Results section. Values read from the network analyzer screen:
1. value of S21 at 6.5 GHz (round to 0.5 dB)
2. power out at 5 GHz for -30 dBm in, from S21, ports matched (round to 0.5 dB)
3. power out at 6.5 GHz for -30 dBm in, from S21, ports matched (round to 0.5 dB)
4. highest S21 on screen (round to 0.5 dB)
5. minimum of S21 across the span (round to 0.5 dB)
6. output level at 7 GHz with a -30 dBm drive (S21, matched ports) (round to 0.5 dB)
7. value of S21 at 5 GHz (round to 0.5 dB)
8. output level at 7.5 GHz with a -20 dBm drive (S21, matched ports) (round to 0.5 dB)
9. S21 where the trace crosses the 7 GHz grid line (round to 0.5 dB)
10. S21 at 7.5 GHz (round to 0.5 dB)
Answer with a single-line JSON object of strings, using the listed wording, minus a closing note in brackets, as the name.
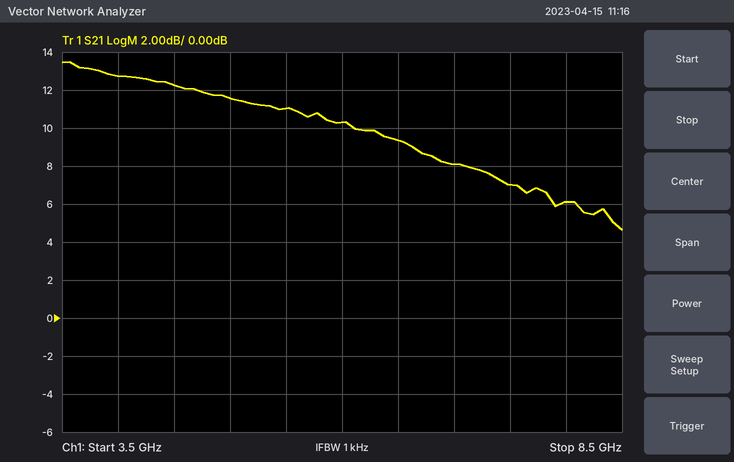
{"value of S21 at 6.5 GHz": "9.5 dB", "power out at 5 GHz for -30 dBm in, from S21, ports matched": "-18.5 dBm", "power out at 6.5 GHz for -30 dBm in, from S21, ports matched": "-20.5 dBm", "highest S21 on screen": "13.5 dB", "minimum of S21 across the span": "4.5 dB", "output level at 7 GHz with a -30 dBm drive (S21, matched ports)": "-22.0 dBm", "value of S21 at 5 GHz": "11.5 dB", "output level at 7.5 GHz with a -20 dBm drive (S21, matched ports)": "-13.0 dBm", "S21 where the trace crosses the 7 GHz grid line": "8.0 dB", "S21 at 7.5 GHz": "7.0 dB"}
